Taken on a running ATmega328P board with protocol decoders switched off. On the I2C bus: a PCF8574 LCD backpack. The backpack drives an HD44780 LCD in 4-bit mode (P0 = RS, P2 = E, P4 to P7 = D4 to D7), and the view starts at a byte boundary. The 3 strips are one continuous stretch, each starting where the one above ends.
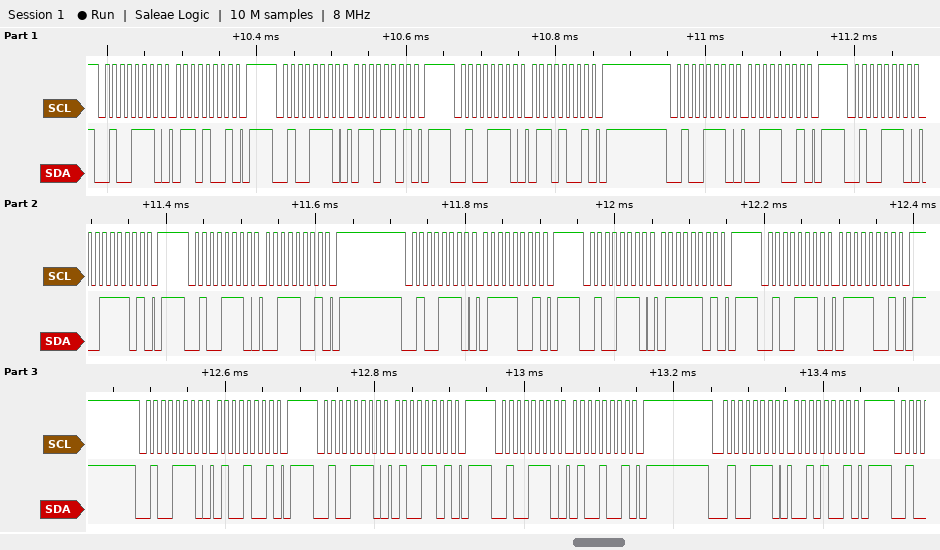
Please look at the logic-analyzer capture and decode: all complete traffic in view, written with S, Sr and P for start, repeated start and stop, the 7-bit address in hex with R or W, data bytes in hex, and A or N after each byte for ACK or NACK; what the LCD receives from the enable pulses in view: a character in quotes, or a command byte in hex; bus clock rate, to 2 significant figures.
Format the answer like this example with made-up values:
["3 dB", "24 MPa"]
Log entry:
["S 27W A 69 A P S 27W A 6D A P S 27W A 69 A P S 27W A 39 A P S 27W A 3D A P S 27W A 39 A P S 27W A 79 A P S 27W A 7D A P S 27W A 79 A P S 27W A 49 A P S 27W A 4D A P S 27W A 49 A P S 27W A 29 A P", "'c' 't'", "100 kHz"]
